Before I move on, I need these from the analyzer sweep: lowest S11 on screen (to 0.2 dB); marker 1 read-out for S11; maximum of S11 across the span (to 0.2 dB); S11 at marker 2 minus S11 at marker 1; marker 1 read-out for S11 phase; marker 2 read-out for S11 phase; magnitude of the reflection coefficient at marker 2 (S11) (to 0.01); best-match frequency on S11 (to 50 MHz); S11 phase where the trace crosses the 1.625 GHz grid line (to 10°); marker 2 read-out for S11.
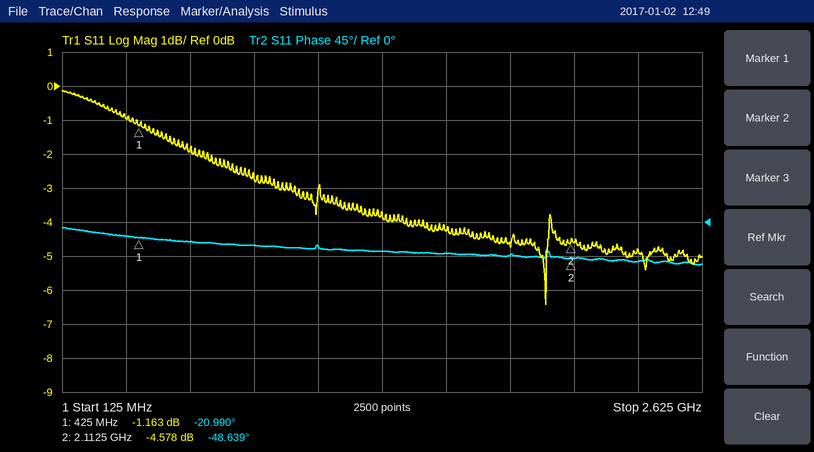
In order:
-6.4 dB
-1.163 dB
-0.2 dB
-3.415 dB
-20.990°
-48.639°
0.59
2.00 GHz
-40°
-4.578 dB
